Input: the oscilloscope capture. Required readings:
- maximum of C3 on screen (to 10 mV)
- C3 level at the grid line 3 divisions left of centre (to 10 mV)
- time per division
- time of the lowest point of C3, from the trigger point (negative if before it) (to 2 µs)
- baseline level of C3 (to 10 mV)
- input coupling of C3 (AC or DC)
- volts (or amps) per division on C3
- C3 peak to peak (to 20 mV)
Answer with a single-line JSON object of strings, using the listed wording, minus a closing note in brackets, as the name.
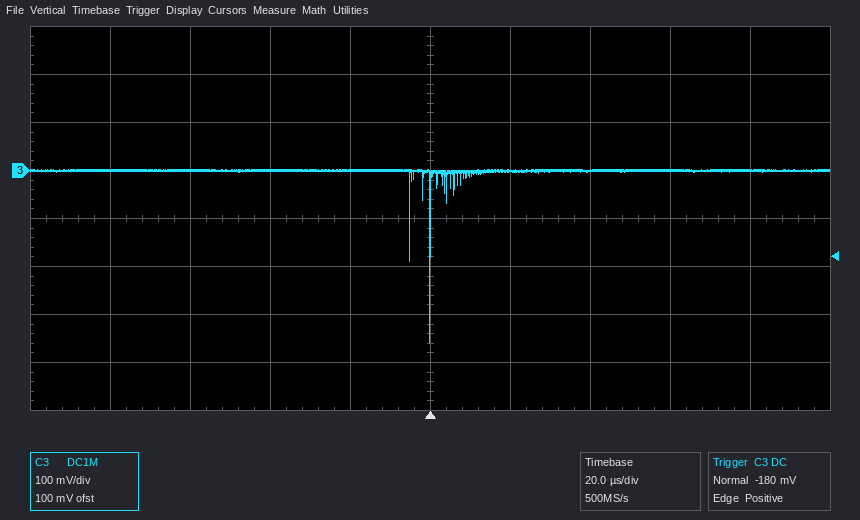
{"maximum of C3 on screen": "0 mV", "C3 level at the grid line 3 divisions left of centre": "0 mV", "time per division": "20 µs", "time of the lowest point of C3, from the trigger point (negative if before it)": "0 µs", "baseline level of C3": "0 mV", "input coupling of C3": "DC", "volts (or amps) per division on C3": "100 mV", "C3 peak to peak": "360 mV"}
